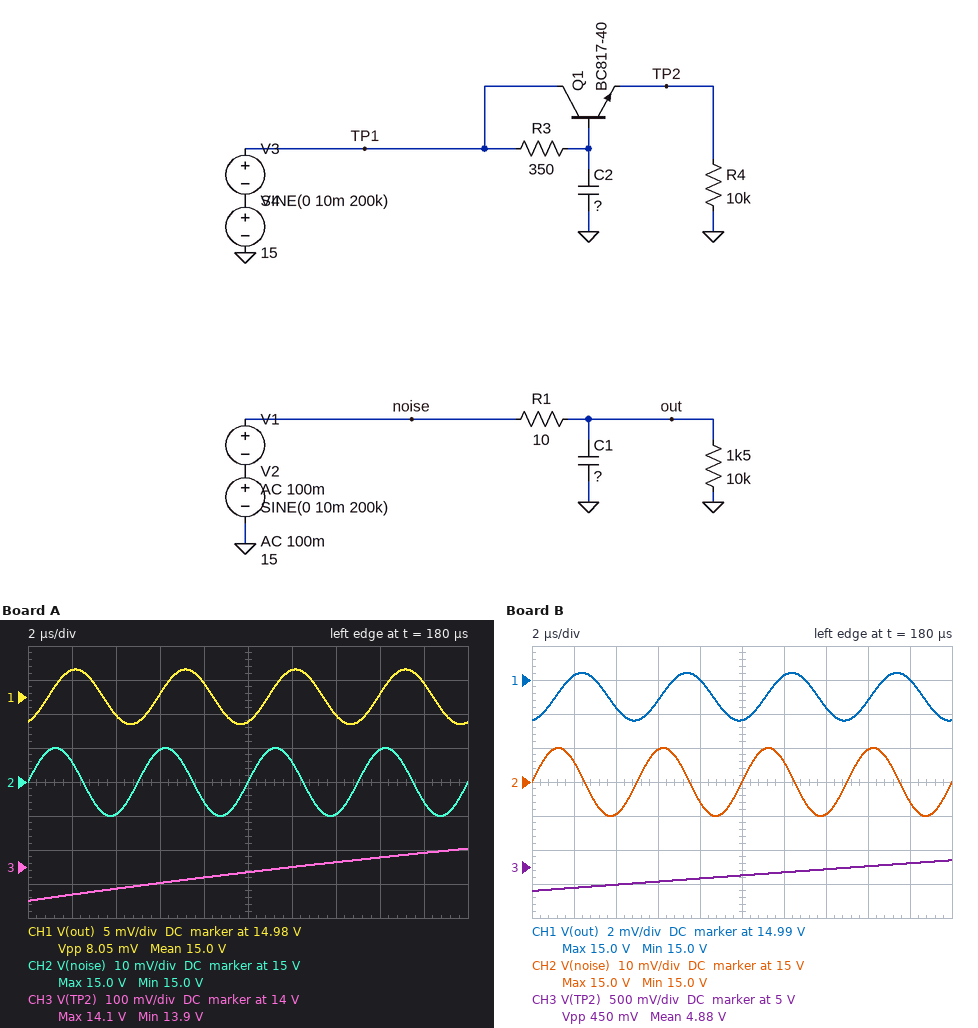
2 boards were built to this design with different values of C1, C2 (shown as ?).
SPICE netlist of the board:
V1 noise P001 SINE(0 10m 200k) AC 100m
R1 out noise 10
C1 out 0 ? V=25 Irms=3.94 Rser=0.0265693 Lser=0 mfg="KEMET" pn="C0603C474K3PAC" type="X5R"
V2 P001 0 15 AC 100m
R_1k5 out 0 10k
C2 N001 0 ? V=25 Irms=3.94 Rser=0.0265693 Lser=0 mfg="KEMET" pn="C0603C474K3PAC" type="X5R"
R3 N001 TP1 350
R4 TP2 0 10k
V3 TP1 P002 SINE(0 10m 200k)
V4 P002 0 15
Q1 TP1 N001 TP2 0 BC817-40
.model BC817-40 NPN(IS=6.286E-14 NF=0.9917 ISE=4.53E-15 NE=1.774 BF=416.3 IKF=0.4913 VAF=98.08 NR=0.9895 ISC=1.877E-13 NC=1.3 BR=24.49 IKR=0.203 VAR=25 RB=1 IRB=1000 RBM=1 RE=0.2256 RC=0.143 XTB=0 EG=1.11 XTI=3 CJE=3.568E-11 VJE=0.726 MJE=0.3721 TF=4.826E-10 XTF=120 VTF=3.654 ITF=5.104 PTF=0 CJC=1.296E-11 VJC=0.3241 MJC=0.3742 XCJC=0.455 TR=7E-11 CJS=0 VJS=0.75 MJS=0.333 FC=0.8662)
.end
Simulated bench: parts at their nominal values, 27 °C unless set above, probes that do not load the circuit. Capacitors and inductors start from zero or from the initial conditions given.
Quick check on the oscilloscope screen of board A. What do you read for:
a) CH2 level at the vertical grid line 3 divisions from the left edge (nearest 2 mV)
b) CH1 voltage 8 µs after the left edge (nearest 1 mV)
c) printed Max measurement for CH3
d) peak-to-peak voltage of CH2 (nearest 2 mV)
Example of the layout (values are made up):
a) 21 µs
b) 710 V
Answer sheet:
a) 15.010 V
b) 14.987 V
c) 14.1 V
d) 20 mV
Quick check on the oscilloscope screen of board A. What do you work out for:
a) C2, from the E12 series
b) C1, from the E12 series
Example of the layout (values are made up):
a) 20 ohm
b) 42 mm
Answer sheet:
a) 150 nF
b) 180 nF
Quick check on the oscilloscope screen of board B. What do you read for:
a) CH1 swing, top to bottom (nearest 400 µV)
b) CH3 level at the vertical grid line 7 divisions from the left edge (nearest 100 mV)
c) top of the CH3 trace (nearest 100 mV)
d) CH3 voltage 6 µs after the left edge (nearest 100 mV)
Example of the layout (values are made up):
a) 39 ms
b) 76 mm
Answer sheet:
a) 2.8 mV
b) 5.0 V
c) 5.1 V
d) 4.8 V
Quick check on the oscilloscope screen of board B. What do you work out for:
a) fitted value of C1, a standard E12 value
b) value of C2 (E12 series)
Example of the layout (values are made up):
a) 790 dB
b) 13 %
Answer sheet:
a) 560 nF
b) 1.2 µF
